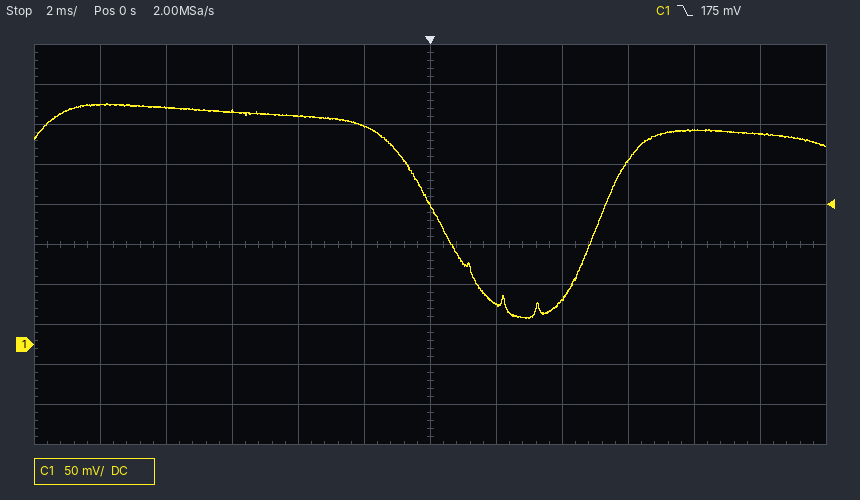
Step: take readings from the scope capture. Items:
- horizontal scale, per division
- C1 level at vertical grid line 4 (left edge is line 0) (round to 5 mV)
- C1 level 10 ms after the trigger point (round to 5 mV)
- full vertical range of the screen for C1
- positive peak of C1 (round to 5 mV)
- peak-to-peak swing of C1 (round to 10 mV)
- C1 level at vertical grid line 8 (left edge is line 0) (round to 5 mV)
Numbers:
2 ms
285 mV
265 mV
500 mV
300 mV
270 mV
55 mV
